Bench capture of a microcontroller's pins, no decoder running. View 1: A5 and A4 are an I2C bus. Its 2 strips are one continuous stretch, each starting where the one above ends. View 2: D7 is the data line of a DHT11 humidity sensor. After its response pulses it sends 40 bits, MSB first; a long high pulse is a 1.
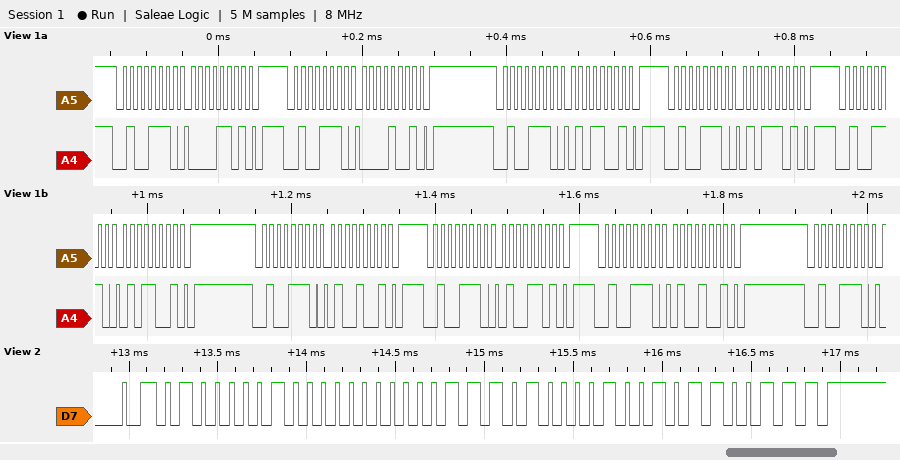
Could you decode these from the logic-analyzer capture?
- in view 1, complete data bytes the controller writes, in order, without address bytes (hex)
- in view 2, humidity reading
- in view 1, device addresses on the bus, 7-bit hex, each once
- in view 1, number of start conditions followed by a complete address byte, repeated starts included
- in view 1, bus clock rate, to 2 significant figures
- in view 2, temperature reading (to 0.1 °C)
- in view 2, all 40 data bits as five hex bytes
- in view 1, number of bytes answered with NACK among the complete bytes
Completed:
0D 09 59 5D 59 49 4D 49
65 %
0x27
9
100 kHz
29.9 °C
41 00 1D 09 67
0
